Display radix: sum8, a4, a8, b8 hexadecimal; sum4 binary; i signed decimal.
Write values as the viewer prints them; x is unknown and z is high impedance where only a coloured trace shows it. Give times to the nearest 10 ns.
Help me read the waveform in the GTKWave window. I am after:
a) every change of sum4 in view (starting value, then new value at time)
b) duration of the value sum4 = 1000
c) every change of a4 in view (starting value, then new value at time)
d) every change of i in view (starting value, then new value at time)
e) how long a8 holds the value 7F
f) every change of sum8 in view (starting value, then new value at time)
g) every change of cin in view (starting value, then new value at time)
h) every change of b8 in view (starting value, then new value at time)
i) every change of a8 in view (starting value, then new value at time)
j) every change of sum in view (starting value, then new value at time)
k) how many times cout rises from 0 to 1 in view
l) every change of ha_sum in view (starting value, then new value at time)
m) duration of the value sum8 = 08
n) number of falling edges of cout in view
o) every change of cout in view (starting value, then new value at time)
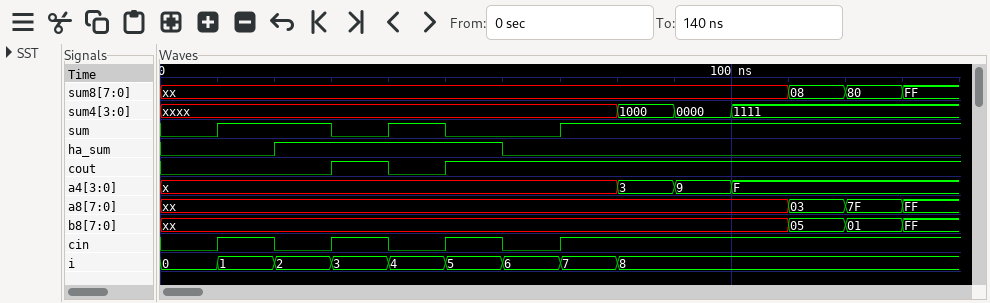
xxxx, 1000 at 80 ns, 0000 at 90 ns, 1111 at 100 ns
10 ns
x, 3 at 80 ns, 9 at 90 ns, F at 100 ns
0, 1 at 10 ns, 2 at 20 ns, 3 at 30 ns, 4 at 40 ns, 5 at 50 ns, 6 at 60 ns, 7 at 70 ns, 8 at 80 ns
10 ns
xx, 08 at 110 ns, 80 at 120 ns, FF at 130 ns
0, 1 at 10 ns, 0 at 20 ns, 1 at 30 ns, 0 at 40 ns, 1 at 50 ns, 0 at 60 ns, 1 at 70 ns
xx, 05 at 110 ns, 01 at 120 ns, FF at 130 ns
xx, 03 at 110 ns, 7F at 120 ns, FF at 130 ns
0, 1 at 10 ns, 0 at 30 ns, 1 at 40 ns, 0 at 50 ns, 1 at 70 ns
2
0, 1 at 20 ns, 0 at 60 ns
10 ns
1
0, 1 at 30 ns, 0 at 40 ns, 1 at 50 ns
